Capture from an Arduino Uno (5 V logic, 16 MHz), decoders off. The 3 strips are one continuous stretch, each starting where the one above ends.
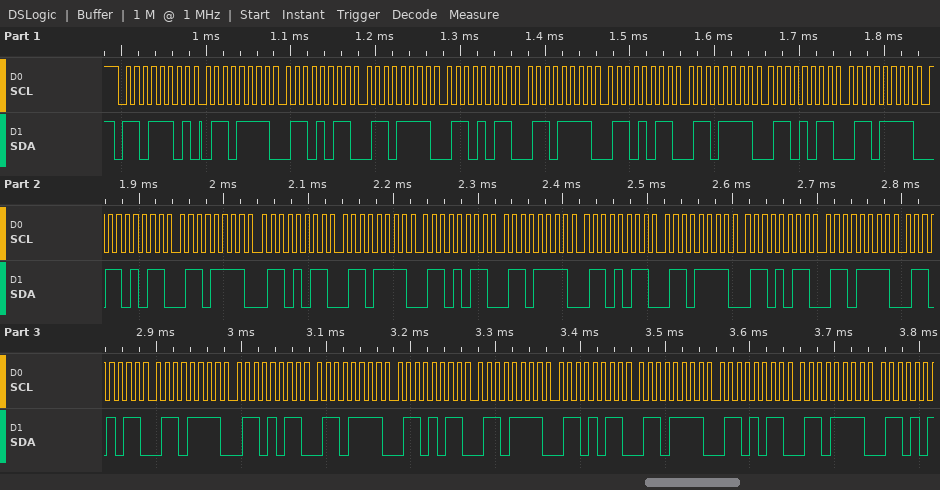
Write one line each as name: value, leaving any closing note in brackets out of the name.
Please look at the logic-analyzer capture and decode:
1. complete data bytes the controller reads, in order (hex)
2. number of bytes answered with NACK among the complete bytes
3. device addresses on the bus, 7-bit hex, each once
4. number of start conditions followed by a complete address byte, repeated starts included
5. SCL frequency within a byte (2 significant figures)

complete data bytes the controller reads, in order: 6F 6B 6F 6B 6F 6B 6F 6B 6F 6B 6F 6B 6F 6B 6F 6B 6F 6B 6F 6B 6F 6B 6F 6B 6F 6B 6F 6B 6F
number of bytes answered with NACK among the complete bytes: 0
device addresses on the bus, 7-bit hex, each once: 0x6E
number of start conditions followed by a complete address byte, repeated starts included: 1
SCL frequency within a byte: 100 kHz
